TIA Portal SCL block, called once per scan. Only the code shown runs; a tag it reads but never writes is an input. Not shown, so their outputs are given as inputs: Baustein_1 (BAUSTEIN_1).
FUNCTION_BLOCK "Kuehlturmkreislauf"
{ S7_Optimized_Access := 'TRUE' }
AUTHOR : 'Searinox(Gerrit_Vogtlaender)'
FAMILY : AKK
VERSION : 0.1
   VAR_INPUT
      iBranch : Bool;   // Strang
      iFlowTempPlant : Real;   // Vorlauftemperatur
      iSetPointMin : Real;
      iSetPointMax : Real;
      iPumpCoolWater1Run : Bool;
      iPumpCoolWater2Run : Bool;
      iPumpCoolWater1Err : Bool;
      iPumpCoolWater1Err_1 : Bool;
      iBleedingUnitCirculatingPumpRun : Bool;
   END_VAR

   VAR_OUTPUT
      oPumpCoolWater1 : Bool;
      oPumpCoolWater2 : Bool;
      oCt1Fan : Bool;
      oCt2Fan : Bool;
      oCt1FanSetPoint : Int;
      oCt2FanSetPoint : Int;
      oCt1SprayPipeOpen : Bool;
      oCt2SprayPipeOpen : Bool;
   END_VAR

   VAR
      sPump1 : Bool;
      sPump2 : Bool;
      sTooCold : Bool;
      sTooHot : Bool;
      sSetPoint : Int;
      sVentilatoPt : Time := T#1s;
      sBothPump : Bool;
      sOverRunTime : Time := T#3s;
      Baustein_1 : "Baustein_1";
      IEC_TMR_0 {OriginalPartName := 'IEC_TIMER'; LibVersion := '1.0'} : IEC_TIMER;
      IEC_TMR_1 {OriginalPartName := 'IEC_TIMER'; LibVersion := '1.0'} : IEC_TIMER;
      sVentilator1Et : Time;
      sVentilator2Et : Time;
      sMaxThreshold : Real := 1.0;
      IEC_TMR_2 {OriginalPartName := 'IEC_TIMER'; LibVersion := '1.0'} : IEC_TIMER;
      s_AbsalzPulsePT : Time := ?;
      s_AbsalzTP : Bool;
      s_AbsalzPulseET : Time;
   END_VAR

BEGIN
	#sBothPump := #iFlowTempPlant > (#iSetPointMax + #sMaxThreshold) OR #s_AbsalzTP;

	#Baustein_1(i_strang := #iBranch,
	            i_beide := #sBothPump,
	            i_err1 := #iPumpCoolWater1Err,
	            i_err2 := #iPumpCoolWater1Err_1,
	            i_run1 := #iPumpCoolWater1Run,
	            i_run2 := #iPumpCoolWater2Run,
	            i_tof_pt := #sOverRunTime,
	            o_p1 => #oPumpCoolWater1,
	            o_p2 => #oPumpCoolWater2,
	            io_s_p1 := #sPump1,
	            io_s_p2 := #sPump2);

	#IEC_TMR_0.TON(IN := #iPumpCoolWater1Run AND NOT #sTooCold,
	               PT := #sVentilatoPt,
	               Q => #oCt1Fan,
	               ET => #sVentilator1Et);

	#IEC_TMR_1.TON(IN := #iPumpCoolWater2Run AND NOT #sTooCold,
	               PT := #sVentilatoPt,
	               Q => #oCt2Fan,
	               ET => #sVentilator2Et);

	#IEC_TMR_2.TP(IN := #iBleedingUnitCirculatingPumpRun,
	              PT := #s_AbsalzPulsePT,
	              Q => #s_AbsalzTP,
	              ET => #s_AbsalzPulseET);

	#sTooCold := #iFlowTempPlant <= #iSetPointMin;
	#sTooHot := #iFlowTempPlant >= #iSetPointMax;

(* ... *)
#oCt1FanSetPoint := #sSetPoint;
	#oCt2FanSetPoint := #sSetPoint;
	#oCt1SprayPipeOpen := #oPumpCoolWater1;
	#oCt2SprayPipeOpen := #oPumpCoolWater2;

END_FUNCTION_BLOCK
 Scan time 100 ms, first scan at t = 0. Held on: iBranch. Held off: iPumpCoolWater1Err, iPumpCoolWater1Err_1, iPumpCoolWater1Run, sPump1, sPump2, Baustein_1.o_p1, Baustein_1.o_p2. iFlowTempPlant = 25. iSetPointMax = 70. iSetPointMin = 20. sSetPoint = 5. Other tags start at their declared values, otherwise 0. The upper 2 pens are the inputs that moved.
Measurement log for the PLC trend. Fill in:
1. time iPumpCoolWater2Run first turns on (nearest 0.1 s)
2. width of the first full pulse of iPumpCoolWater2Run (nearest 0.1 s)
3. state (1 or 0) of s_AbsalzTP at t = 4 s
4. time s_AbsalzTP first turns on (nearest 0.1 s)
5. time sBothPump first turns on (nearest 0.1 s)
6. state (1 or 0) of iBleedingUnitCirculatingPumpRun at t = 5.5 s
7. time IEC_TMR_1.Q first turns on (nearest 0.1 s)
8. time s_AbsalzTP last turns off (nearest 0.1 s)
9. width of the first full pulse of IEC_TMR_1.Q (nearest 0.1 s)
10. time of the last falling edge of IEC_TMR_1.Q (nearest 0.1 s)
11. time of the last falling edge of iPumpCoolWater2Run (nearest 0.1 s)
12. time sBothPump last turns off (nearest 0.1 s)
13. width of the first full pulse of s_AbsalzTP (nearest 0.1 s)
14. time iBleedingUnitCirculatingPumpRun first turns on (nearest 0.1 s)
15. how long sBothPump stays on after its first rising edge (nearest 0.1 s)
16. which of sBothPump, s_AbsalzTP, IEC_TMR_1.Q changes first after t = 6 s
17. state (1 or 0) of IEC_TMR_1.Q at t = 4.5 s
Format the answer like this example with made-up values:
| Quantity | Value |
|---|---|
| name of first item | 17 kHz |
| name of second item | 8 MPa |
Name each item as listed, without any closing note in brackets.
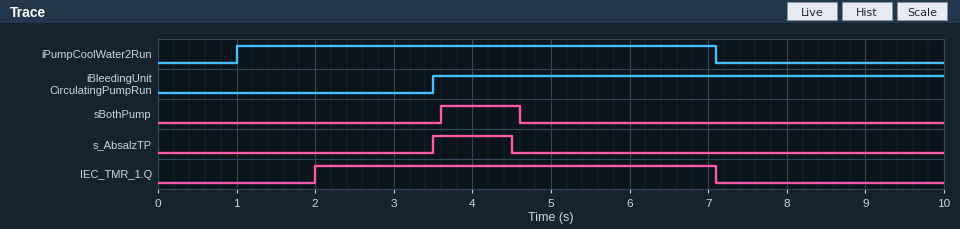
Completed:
| Quantity | Value |
|---|---|
| time iPumpCoolWater2Run first turns on | 1.0 s |
| width of the first full pulse of iPumpCoolWater2Run | 6.1 s |
| state (1 or 0) of s_AbsalzTP at t = 4 s | 1 |
| time s_AbsalzTP first turns on | 3.5 s |
| time sBothPump first turns on | 3.6 s |
| state (1 or 0) of iBleedingUnitCirculatingPumpRun at t = 5.5 s | 1 |
| time IEC_TMR_1.Q first turns on | 2.0 s |
| time s_AbsalzTP last turns off | 4.5 s |
| width of the first full pulse of IEC_TMR_1.Q | 5.1 s |
| time of the last falling edge of IEC_TMR_1.Q | 7.1 s |
| time of the last falling edge of iPumpCoolWater2Run | 7.1 s |
| time sBothPump last turns off | 4.6 s |
| width of the first full pulse of s_AbsalzTP | 1.0 s |
| time iBleedingUnitCirculatingPumpRun first turns on | 3.5 s |
| how long sBothPump stays on after its first rising edge | 1.0 s |
| which of sBothPump, s_AbsalzTP, IEC_TMR_1.Q changes first after t = 6 s | IEC_TMR_1.Q |
| state (1 or 0) of IEC_TMR_1.Q at t = 4.5 s | 1 |
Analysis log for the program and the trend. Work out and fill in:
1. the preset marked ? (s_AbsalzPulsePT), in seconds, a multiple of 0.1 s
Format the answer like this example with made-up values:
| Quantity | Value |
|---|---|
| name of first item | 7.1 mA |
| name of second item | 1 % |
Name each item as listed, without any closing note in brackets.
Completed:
| Quantity | Value |
|---|---|
| the preset marked ? (s_AbsalzPulsePT), in seconds, a multiple of 0.1 s | 1.0 s |
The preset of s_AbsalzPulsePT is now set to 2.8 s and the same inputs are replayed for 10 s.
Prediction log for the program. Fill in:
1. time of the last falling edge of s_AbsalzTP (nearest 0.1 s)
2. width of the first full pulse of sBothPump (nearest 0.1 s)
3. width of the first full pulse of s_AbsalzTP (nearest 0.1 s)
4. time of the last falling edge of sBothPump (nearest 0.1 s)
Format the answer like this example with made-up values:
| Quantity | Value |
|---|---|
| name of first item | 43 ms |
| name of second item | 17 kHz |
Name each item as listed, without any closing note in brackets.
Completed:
| Quantity | Value |
|---|---|
| time of the last falling edge of s_AbsalzTP | 6.3 s |
| width of the first full pulse of sBothPump | 2.8 s |
| width of the first full pulse of s_AbsalzTP | 2.8 s |
| time of the last falling edge of sBothPump | 6.4 s |
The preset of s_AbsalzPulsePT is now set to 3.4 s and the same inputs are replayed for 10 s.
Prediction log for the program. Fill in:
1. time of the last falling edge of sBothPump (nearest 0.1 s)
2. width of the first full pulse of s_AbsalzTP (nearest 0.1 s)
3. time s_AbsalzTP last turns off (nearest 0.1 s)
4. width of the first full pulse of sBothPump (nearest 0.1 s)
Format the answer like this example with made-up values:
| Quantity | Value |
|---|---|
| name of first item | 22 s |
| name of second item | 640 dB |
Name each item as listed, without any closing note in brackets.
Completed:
| Quantity | Value |
|---|---|
| time of the last falling edge of sBothPump | 7.0 s |
| width of the first full pulse of s_AbsalzTP | 3.4 s |
| time s_AbsalzTP last turns off | 6.9 s |
| width of the first full pulse of sBothPump | 3.4 s |
